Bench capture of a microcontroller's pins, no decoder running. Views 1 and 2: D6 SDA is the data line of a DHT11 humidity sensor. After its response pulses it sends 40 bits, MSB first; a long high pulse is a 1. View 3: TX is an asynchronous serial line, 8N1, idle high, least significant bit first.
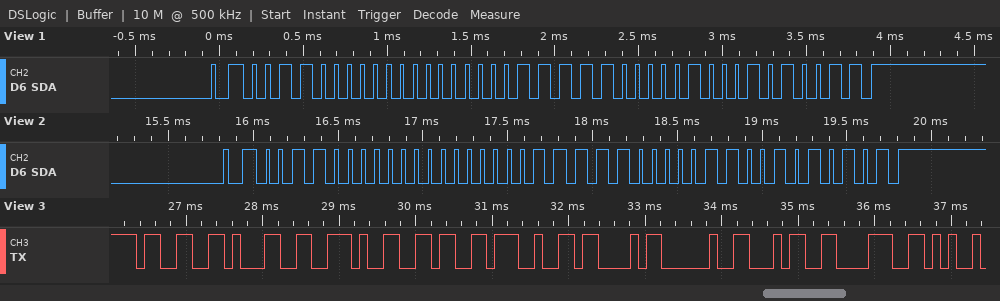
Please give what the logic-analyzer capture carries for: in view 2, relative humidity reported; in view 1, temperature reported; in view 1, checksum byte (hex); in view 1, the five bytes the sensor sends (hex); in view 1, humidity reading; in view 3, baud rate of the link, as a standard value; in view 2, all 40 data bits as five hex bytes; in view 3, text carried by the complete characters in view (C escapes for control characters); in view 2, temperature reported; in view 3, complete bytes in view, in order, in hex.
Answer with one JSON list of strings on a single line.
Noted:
["48 %", "31.4 °C", "0x53", "30 00 1F 04 53", "48 %", "9600 baud", "30 00 1F 06 55", "\"31.6'C 48\"", "31.6 °C", "33 31 2E 36 27 43 20 34 38"]
